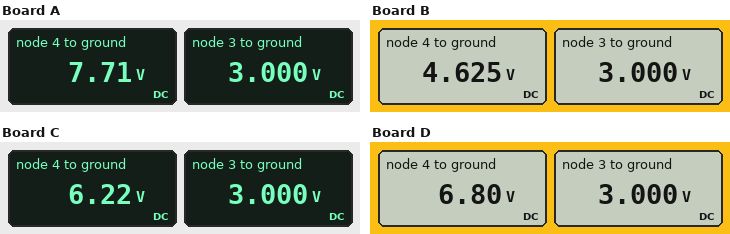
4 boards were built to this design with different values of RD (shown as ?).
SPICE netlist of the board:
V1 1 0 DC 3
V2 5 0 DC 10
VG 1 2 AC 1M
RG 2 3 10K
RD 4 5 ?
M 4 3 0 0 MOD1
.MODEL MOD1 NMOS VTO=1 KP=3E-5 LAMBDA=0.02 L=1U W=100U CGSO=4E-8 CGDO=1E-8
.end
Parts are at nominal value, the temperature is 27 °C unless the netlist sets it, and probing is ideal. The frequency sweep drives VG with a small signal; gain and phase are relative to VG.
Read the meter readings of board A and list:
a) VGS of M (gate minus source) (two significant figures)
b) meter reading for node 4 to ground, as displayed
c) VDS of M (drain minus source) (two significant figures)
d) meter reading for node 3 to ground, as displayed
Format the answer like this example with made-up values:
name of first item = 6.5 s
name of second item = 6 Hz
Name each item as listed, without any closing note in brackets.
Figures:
VGS of M (gate minus source) = 3.0 V
meter reading for node 4 to ground, as displayed = 7.71 V
VDS of M (drain minus source) = 7.7 V
meter reading for node 3 to ground, as displayed = 3.000 V
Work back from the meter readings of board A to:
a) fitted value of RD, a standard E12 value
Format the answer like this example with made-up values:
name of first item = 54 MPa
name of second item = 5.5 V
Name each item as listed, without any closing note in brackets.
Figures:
fitted value of RD, a standard E12 value = 330 Ω
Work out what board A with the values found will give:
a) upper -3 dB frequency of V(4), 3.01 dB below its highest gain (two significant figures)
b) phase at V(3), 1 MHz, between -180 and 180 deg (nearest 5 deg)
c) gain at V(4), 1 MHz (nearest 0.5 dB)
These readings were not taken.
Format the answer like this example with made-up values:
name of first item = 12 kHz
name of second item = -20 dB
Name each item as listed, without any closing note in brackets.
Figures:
upper -3 dB frequency of V(4), 3.01 dB below its highest gain = 2.2 MHz
phase at V(3), 1 MHz, between -180 and 180 deg = 155 deg
gain at V(4), 1 MHz = 6.0 dB
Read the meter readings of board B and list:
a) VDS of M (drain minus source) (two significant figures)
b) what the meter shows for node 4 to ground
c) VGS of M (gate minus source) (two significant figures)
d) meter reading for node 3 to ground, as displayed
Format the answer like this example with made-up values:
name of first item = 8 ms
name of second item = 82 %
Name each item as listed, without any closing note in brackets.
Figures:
VDS of M (drain minus source) = 4.6 V
what the meter shows for node 4 to ground = 4.625 V
VGS of M (gate minus source) = 3.0 V
meter reading for node 3 to ground, as displayed = 3.000 V
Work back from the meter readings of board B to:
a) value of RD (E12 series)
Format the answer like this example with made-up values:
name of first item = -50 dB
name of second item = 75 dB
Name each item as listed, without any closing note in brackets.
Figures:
value of RD = 820 Ω
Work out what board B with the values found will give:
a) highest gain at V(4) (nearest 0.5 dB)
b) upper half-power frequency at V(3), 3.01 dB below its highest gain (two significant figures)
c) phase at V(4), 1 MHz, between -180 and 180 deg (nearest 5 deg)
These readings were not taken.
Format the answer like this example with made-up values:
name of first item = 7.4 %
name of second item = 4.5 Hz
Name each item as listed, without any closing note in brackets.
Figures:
highest gain at V(4) = 14.0 dB
upper half-power frequency at V(3), 3.01 dB below its highest gain = 1.6 MHz
phase at V(4), 1 MHz, between -180 and 180 deg = -30 deg
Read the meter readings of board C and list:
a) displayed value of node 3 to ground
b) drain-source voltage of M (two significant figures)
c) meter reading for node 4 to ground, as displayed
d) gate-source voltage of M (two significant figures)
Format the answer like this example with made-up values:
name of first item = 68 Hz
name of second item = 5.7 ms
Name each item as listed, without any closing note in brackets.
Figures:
displayed value of node 3 to ground = 3.000 V
drain-source voltage of M = 6.2 V
meter reading for node 4 to ground, as displayed = 6.22 V
gate-source voltage of M = 3.0 V
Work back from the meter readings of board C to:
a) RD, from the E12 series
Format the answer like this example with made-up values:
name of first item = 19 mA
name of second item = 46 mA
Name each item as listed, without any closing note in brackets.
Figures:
RD, from the E12 series = 560 Ω
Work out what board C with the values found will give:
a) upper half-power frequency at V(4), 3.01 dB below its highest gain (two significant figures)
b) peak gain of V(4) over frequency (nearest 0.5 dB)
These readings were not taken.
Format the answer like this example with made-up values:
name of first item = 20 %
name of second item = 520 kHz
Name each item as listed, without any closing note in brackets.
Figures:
upper half-power frequency at V(4), 3.01 dB below its highest gain = 1.9 MHz
peak gain of V(4) over frequency = 11.0 dB
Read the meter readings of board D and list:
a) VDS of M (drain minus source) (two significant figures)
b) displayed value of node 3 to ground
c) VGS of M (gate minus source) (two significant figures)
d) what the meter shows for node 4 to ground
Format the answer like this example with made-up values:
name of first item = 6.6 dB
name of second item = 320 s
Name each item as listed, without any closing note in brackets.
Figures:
VDS of M (drain minus source) = 6.8 V
displayed value of node 3 to ground = 3.000 V
VGS of M (gate minus source) = 3.0 V
what the meter shows for node 4 to ground = 6.80 V
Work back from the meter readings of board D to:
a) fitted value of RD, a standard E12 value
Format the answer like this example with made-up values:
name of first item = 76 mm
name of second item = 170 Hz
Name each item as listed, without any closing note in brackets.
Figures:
fitted value of RD, a standard E12 value = 470 Ω
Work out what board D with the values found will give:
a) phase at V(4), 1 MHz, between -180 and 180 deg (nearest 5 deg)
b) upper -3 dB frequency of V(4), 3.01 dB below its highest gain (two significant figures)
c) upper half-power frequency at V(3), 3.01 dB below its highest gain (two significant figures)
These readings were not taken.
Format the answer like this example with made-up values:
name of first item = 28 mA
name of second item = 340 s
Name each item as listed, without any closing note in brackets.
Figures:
phase at V(4), 1 MHz, between -180 and 180 deg = -25 deg
upper -3 dB frequency of V(4), 3.01 dB below its highest gain = 2.0 MHz
upper half-power frequency at V(3), 3.01 dB below its highest gain = 2.0 MHz
